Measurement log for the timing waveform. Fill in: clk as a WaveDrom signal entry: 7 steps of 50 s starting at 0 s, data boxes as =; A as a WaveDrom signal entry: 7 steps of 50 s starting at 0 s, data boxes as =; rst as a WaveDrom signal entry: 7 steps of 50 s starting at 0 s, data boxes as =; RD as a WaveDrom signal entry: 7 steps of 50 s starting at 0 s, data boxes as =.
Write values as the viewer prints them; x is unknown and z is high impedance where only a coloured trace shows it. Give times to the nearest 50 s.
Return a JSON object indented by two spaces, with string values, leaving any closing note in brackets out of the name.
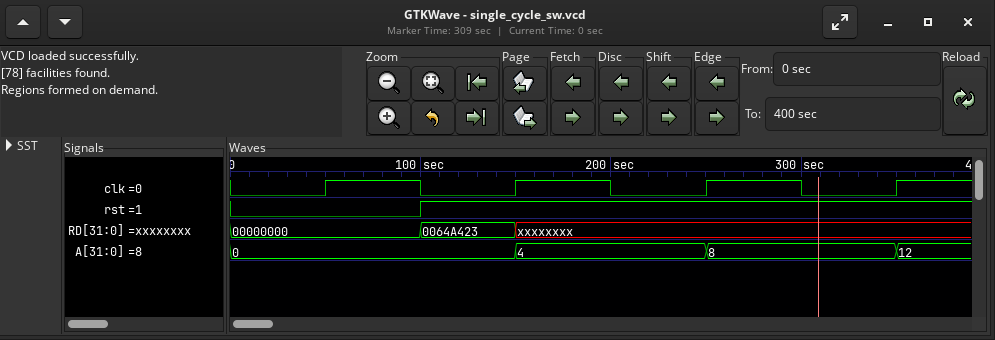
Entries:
{
  "clk as a WaveDrom signal entry: 7 steps of 50 s starting at 0 s, data boxes as =": "{name: 'clk', wave: '0101010'}",
  "A as a WaveDrom signal entry: 7 steps of 50 s starting at 0 s, data boxes as =": "{name: 'A', wave: '=..=.=.', data: '0 4 8'}",
  "rst as a WaveDrom signal entry: 7 steps of 50 s starting at 0 s, data boxes as =": "{name: 'rst', wave: '0.1....'}",
  "RD as a WaveDrom signal entry: 7 steps of 50 s starting at 0 s, data boxes as =": "{name: 'RD', wave: '=.=x...', data: '00000000 0064A423'}"
}
